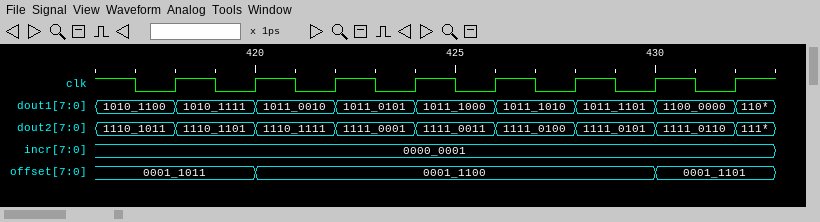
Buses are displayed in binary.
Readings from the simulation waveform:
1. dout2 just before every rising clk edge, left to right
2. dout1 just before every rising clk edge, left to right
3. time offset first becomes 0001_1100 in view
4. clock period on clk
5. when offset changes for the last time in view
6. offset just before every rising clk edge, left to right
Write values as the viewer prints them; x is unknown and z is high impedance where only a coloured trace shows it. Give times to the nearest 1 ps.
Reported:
1110_1011, 1110_1101, 1110_1111, 1111_0001, 1111_0011, 1111_0100, 1111_0101, 1111_0110
1010_1100, 1010_1111, 1011_0010, 1011_0101, 1011_1000, 1011_1010, 1011_1101, 1100_0000
420 ps
2 ps
430 ps
0001_1011, 0001_1011, 0001_1100, 0001_1100, 0001_1100, 0001_1100, 0001_1100, 0001_1101
